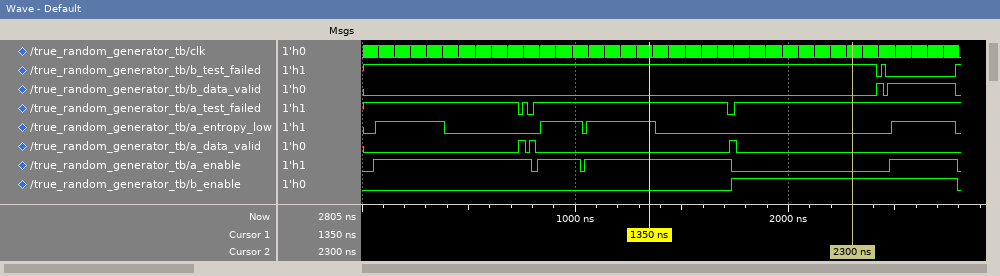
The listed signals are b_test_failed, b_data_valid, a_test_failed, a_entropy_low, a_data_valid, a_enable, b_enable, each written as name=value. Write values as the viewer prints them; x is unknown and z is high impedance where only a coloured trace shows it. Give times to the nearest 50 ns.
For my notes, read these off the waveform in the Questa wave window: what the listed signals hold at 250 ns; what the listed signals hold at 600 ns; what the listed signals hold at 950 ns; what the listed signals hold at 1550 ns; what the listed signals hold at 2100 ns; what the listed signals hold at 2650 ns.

b_test_failed=1, b_data_valid=0, a_test_failed=1, a_entropy_low=1, a_data_valid=0, a_enable=1, b_enable=0
b_test_failed=1, b_data_valid=0, a_test_failed=1, a_entropy_low=0, a_data_valid=0, a_enable=1, b_enable=0
b_test_failed=1, b_data_valid=0, a_test_failed=1, a_entropy_low=1, a_data_valid=0, a_enable=1, b_enable=0
b_test_failed=1, b_data_valid=0, a_test_failed=1, a_entropy_low=0, a_data_valid=0, a_enable=1, b_enable=0
b_test_failed=1, b_data_valid=0, a_test_failed=1, a_entropy_low=0, a_data_valid=0, a_enable=0, b_enable=1
b_test_failed=0, b_data_valid=1, a_test_failed=1, a_entropy_low=1, a_data_valid=0, a_enable=1, b_enable=1
